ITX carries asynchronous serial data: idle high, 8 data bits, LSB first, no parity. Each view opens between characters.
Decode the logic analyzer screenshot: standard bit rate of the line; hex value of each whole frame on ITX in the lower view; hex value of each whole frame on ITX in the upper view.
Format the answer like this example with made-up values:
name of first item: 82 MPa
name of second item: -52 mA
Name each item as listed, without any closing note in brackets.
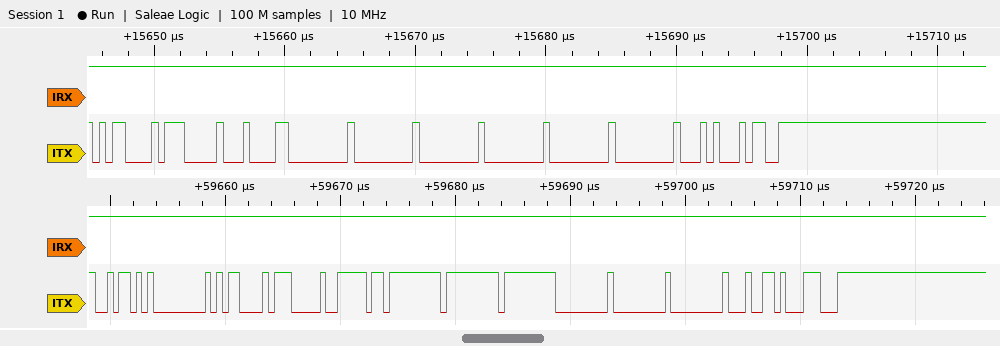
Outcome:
standard bit rate of the line: 2000000 baud
hex value of each whole frame on ITX in the lower view: 5A, 00, 0D, 07, BE, FF, FF, FF, 00, 00, 00, 64, 1C
hex value of each whole frame on ITX in the upper view: 0D, 07, 84, 00, 00, 00, 00, 00, 00, 14, F3
